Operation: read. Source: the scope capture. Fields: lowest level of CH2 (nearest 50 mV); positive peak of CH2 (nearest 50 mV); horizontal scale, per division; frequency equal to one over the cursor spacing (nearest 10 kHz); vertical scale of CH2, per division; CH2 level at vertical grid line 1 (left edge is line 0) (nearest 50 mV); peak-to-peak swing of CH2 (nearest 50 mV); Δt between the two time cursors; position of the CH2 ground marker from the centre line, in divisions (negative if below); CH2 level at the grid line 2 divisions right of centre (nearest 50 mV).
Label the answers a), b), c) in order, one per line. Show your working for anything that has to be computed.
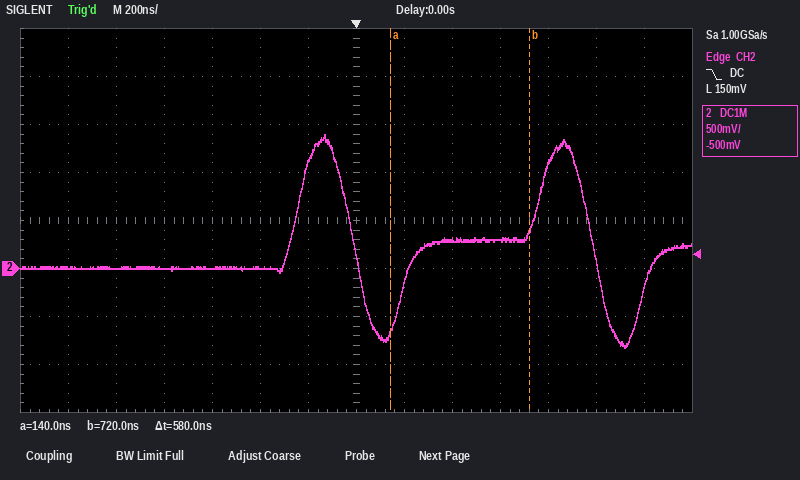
a) -800 mV
b) 1.40 V
c) 200 ns
d) 1 / 580 ns ≈ 1.72 MHz
e) 500 mV
f) 0 mV
g) 1.40 V − (-800 mV) = 2.20 V
h) 580 ns
i) -1.0 div
j) 300 mV
